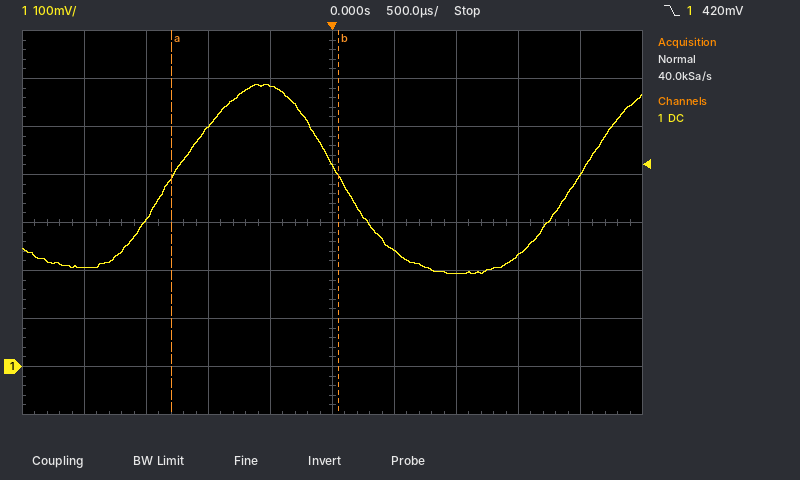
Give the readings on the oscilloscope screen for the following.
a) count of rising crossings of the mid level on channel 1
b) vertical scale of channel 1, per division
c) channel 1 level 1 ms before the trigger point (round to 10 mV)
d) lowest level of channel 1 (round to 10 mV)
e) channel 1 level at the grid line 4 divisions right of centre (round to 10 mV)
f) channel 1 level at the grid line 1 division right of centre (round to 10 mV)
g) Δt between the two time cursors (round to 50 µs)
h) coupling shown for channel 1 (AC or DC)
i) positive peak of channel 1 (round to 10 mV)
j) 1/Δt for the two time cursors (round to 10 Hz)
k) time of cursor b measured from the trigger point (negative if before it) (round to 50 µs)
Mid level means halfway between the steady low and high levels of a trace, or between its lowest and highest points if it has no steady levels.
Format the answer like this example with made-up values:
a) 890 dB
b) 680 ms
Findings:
a) 2
b) 100 mV
c) 500 mV
d) 190 mV
e) 400 mV
f) 240 mV
g) 1.35 ms
h) DC
i) 590 mV
j) 740 Hz
k) +50 µs
